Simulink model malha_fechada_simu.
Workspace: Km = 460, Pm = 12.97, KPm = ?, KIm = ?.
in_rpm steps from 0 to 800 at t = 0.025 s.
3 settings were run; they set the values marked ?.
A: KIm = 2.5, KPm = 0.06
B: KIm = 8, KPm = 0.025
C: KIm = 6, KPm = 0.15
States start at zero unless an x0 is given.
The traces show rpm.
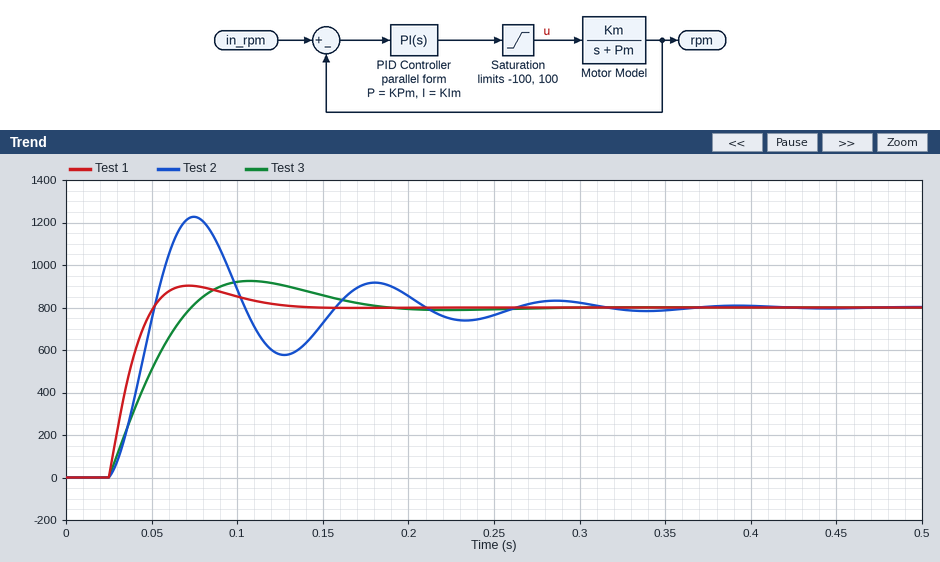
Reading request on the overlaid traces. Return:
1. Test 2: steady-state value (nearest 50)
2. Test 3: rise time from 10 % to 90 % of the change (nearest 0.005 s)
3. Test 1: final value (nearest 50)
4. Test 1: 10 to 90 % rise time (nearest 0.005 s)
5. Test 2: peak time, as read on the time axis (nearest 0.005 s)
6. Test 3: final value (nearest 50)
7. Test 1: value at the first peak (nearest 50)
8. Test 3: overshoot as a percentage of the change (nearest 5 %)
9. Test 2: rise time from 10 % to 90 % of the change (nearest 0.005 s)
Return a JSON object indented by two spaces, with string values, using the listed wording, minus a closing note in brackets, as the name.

{
  "Test 2: steady-state value": "800",
  "Test 3: rise time from 10 % to 90 % of the change": "0.035 s",
  "Test 1: final value": "800",
  "Test 1: 10 to 90 % rise time": "0.020 s",
  "Test 2: peak time, as read on the time axis": "0.075 s",
  "Test 3: final value": "800",
  "Test 1: value at the first peak": "900",
  "Test 3: overshoot as a percentage of the change": "15 %",
  "Test 2: rise time from 10 % to 90 % of the change": "0.020 s"
}
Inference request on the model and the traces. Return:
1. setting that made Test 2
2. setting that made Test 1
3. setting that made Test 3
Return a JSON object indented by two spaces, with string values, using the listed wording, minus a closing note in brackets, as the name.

{
  "setting that made Test 2": "B",
  "setting that made Test 1": "C",
  "setting that made Test 3": "A"
}
